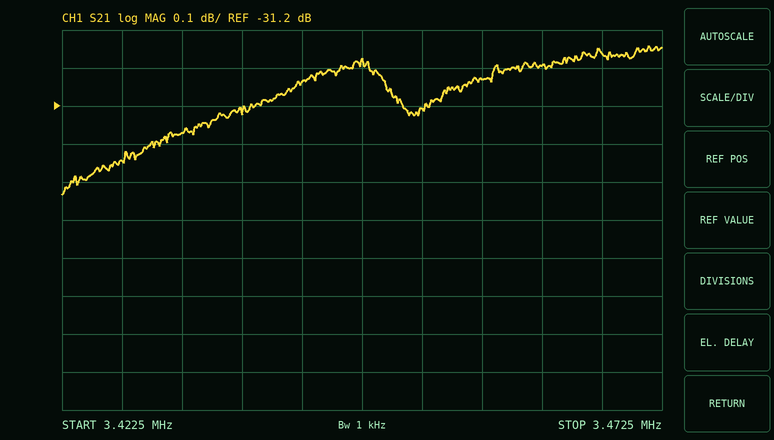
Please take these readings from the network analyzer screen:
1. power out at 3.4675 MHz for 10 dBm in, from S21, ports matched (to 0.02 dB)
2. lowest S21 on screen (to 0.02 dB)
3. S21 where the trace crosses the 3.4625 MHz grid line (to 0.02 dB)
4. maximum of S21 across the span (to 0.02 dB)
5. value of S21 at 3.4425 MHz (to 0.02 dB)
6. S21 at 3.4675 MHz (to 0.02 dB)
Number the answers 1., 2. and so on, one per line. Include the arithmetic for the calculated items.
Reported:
1. 10 dBm + (-31.06 dB) = -21.06 dBm
2. -31.44 dB
3. -31.10 dB
4. -31.04 dB
5. -31.14 dB
6. -31.06 dB
